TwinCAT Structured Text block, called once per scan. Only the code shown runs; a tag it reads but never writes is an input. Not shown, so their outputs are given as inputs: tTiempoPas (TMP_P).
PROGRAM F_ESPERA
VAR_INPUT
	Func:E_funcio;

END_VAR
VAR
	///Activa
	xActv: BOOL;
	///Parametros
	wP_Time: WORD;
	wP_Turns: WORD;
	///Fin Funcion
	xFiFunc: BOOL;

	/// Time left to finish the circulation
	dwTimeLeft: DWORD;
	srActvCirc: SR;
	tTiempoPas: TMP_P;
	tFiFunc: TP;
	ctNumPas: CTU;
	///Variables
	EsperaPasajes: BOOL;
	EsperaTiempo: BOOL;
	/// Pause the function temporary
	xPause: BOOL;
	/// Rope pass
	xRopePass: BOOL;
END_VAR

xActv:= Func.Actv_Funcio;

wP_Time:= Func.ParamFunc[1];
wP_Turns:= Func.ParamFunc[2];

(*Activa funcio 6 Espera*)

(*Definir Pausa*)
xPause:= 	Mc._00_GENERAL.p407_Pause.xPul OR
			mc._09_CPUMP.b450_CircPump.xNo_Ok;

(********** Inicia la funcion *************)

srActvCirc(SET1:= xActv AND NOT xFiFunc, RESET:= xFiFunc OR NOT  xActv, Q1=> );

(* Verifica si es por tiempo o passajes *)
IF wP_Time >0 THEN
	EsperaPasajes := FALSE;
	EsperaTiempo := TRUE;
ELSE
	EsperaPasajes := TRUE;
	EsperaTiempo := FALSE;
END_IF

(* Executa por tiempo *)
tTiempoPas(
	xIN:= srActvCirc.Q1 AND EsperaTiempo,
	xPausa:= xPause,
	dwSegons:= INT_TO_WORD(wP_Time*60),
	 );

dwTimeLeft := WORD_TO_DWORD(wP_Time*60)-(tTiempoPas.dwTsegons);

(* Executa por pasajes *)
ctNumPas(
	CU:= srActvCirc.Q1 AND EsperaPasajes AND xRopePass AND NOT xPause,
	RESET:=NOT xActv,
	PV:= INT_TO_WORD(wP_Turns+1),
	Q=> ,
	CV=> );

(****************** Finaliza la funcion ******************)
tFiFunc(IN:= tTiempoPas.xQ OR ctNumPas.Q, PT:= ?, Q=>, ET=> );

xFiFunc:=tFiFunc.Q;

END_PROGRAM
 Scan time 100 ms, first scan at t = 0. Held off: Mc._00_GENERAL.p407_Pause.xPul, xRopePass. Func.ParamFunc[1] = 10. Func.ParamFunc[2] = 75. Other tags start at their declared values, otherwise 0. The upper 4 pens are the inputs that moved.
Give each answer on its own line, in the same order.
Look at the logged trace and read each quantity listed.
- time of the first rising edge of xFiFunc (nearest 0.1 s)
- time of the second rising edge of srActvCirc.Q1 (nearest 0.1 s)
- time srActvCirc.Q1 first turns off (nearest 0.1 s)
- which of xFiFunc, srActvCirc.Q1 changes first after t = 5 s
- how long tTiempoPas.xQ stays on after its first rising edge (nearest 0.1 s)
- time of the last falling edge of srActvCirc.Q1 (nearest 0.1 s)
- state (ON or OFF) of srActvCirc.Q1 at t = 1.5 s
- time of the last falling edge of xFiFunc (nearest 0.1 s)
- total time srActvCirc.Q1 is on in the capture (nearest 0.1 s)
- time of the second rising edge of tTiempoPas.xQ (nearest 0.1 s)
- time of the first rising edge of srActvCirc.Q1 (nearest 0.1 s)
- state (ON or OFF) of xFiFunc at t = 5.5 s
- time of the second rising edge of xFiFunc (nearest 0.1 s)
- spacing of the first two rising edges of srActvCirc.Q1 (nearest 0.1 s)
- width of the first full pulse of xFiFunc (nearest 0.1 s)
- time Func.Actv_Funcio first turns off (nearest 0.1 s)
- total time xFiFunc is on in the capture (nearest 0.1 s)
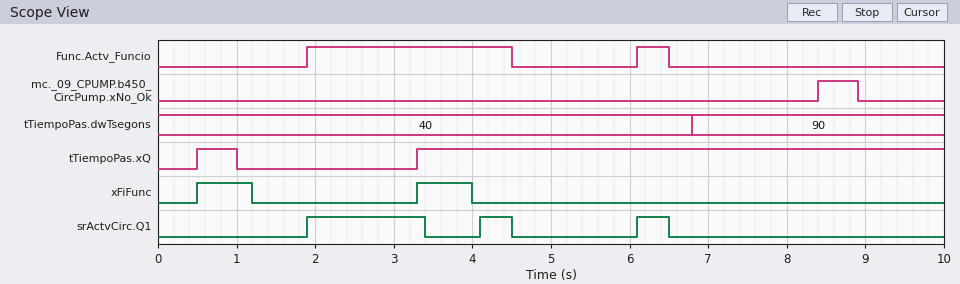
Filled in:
0.5 s
4.1 s
3.4 s
srActvCirc.Q1
0.5 s
6.5 s
OFF
4.0 s
2.3 s
3.3 s
1.9 s
OFF
3.3 s
2.2 s
0.7 s
4.5 s
1.4 s
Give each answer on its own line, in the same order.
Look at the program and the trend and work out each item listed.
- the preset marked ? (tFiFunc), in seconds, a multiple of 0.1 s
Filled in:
0.7 s
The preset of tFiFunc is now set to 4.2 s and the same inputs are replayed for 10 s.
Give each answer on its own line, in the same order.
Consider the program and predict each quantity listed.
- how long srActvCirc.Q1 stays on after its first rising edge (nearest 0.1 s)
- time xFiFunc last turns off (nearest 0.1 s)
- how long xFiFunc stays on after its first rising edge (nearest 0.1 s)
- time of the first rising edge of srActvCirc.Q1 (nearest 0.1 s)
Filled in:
0.4 s
4.7 s
4.2 s
6.1 s
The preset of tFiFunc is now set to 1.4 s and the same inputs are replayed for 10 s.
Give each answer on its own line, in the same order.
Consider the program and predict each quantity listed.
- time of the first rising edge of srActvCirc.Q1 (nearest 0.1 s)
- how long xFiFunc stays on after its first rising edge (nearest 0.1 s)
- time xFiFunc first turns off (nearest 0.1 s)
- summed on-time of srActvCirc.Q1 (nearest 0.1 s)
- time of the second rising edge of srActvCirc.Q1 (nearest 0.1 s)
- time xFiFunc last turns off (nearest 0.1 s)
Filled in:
2.0 s
1.4 s
1.9 s
1.8 s
6.1 s
4.7 s
